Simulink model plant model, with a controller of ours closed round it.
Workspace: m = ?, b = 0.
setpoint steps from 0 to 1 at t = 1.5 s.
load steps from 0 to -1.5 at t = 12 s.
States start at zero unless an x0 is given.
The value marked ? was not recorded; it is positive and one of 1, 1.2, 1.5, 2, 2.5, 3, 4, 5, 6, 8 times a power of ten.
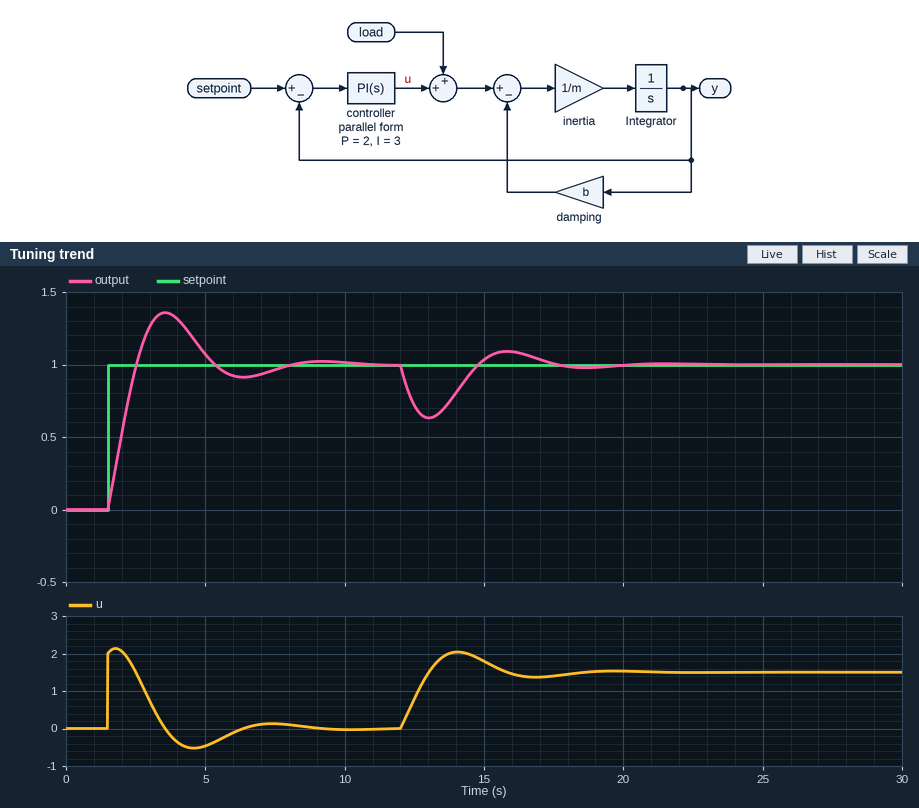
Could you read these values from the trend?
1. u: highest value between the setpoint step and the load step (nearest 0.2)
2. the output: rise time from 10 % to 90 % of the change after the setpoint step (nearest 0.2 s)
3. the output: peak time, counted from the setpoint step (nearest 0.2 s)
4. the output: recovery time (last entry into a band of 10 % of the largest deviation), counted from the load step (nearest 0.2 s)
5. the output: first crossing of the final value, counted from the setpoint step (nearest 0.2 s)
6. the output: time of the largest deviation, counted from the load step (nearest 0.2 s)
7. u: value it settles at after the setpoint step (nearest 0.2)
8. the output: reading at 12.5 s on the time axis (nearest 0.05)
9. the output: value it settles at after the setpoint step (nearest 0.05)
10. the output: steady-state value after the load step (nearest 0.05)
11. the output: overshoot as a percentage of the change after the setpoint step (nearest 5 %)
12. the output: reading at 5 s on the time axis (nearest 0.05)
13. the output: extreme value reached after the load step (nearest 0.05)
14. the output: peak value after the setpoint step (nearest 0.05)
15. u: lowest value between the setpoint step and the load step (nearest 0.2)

2.2
0.8 s
2.0 s
5.0 s
1.0 s
1.0 s
0.0
0.70
1.00
1.00
35 %
1.05
0.65
1.35
-0.6
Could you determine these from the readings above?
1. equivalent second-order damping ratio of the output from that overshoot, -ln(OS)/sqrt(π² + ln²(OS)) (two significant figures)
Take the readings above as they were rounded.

0.32
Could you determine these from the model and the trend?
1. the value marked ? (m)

2
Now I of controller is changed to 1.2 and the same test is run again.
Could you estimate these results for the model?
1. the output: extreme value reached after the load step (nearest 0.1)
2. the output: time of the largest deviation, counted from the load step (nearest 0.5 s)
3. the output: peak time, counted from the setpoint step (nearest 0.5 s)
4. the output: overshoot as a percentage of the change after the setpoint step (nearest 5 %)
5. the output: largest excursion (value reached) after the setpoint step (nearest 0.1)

0.5
1.5 s
3.0 s
25 %
1.2
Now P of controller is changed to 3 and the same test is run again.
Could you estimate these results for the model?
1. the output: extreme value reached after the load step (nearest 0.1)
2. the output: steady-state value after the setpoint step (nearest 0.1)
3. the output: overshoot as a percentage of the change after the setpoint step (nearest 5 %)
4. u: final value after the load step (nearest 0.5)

0.7
1.0
25 %
1.5
